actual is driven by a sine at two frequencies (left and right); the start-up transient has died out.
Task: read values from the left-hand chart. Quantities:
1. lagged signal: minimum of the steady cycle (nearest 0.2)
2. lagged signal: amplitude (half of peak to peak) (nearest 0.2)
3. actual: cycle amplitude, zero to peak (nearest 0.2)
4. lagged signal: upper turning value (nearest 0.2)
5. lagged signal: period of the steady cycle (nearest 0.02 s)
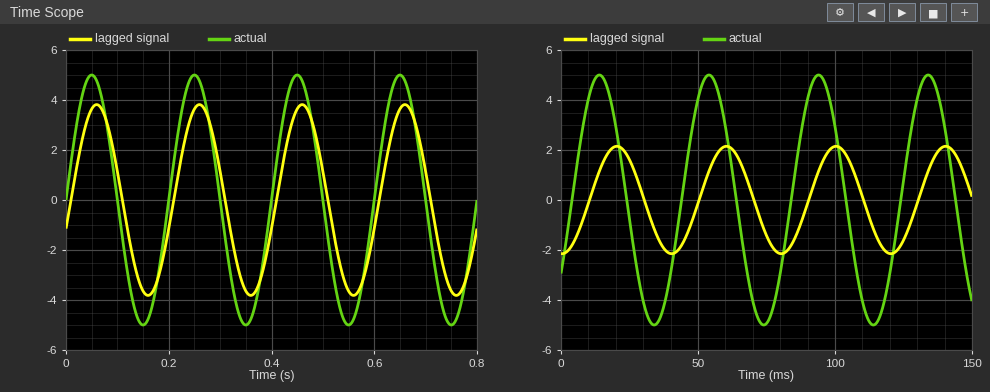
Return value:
-3.8
3.8
5.0
3.8
0.20 s
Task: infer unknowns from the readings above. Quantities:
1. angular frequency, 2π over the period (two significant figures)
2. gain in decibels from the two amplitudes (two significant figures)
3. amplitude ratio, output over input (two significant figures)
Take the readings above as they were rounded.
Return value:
31 rad/s
-2.4 dB
0.76
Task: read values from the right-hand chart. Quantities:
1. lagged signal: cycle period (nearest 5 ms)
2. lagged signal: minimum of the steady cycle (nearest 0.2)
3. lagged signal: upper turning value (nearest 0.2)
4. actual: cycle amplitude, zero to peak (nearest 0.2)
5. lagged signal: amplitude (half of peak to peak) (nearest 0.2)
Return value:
40 ms
-2.2
2.2
5.0
2.2
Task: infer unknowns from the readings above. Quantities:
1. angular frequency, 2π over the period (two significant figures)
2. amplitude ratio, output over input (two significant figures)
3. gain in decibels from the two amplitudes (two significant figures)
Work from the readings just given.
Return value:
0.16 rad/ms
0.44
-7.1 dB
